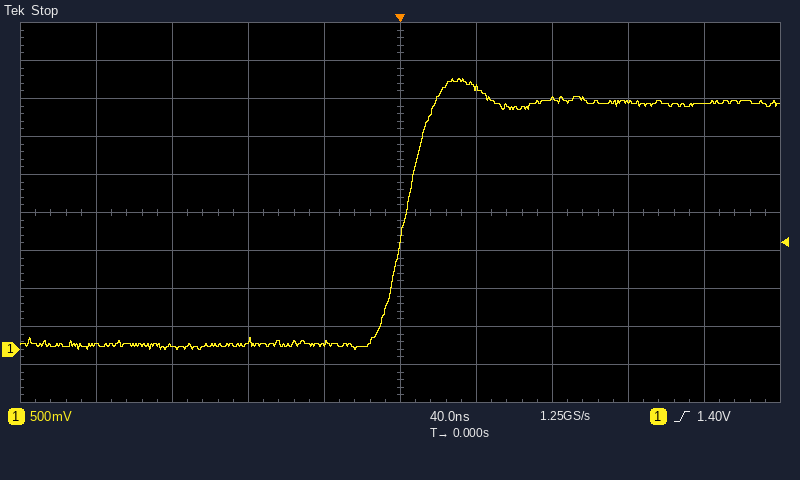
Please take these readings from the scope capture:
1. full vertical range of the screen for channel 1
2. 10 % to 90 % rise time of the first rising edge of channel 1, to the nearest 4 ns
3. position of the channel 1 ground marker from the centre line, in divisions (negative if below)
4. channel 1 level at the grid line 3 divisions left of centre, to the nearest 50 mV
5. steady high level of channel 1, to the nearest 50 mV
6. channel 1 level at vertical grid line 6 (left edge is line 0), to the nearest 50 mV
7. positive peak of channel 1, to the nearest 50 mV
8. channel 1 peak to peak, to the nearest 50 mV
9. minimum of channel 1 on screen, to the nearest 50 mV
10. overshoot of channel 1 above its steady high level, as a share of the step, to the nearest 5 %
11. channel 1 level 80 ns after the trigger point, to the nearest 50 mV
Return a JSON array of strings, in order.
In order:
["5 V", "24 ns", "-3.6 div", "50 mV", "3.25 V", "3.45 V", "3.55 V", "3.55 V", "0 mV", "10 %", "3.30 V"]
